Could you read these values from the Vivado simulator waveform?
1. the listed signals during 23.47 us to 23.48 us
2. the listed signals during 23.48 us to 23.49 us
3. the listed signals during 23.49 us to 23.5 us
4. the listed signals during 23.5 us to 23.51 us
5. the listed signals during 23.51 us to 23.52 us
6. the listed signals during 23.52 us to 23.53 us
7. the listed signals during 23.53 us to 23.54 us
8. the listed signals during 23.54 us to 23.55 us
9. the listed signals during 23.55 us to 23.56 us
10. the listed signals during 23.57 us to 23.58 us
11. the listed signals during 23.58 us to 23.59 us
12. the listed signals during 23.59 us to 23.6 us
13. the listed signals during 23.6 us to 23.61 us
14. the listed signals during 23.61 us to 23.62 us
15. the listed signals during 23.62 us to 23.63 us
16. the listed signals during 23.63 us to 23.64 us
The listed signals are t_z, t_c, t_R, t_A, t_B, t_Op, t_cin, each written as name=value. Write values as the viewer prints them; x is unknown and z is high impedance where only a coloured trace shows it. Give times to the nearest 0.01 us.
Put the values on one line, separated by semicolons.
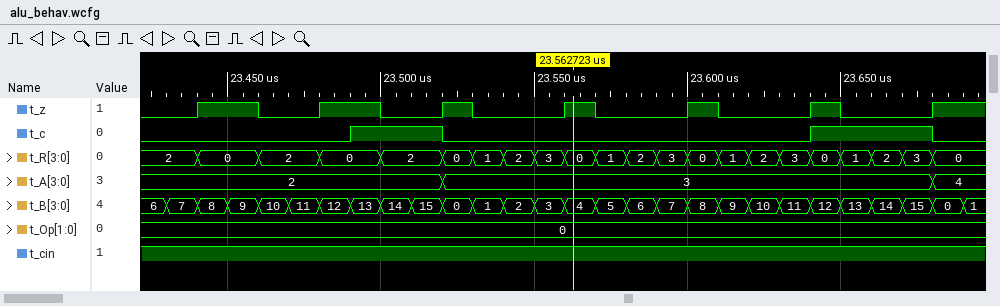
t_z=0, t_c=0, t_R=2, t_A=2, t_B=11, t_Op=0, t_cin=1; t_z=1, t_c=0, t_R=0, t_A=2, t_B=12, t_Op=0, t_cin=1; t_z=1, t_c=1, t_R=0, t_A=2, t_B=13, t_Op=0, t_cin=1; t_z=0, t_c=1, t_R=2, t_A=2, t_B=14, t_Op=0, t_cin=1; t_z=0, t_c=1, t_R=2, t_A=2, t_B=15, t_Op=0, t_cin=1; t_z=1, t_c=0, t_R=0, t_A=3, t_B=0, t_Op=0, t_cin=1; t_z=0, t_c=0, t_R=1, t_A=3, t_B=1, t_Op=0, t_cin=1; t_z=0, t_c=0, t_R=2, t_A=3, t_B=2, t_Op=0, t_cin=1; t_z=0, t_c=0, t_R=3, t_A=3, t_B=3, t_Op=0, t_cin=1; t_z=0, t_c=0, t_R=1, t_A=3, t_B=5, t_Op=0, t_cin=1; t_z=0, t_c=0, t_R=2, t_A=3, t_B=6, t_Op=0, t_cin=1; t_z=0, t_c=0, t_R=3, t_A=3, t_B=7, t_Op=0, t_cin=1; t_z=1, t_c=0, t_R=0, t_A=3, t_B=8, t_Op=0, t_cin=1; t_z=0, t_c=0, t_R=1, t_A=3, t_B=9, t_Op=0, t_cin=1; t_z=0, t_c=0, t_R=2, t_A=3, t_B=10, t_Op=0, t_cin=1; t_z=0, t_c=0, t_R=3, t_A=3, t_B=11, t_Op=0, t_cin=1
